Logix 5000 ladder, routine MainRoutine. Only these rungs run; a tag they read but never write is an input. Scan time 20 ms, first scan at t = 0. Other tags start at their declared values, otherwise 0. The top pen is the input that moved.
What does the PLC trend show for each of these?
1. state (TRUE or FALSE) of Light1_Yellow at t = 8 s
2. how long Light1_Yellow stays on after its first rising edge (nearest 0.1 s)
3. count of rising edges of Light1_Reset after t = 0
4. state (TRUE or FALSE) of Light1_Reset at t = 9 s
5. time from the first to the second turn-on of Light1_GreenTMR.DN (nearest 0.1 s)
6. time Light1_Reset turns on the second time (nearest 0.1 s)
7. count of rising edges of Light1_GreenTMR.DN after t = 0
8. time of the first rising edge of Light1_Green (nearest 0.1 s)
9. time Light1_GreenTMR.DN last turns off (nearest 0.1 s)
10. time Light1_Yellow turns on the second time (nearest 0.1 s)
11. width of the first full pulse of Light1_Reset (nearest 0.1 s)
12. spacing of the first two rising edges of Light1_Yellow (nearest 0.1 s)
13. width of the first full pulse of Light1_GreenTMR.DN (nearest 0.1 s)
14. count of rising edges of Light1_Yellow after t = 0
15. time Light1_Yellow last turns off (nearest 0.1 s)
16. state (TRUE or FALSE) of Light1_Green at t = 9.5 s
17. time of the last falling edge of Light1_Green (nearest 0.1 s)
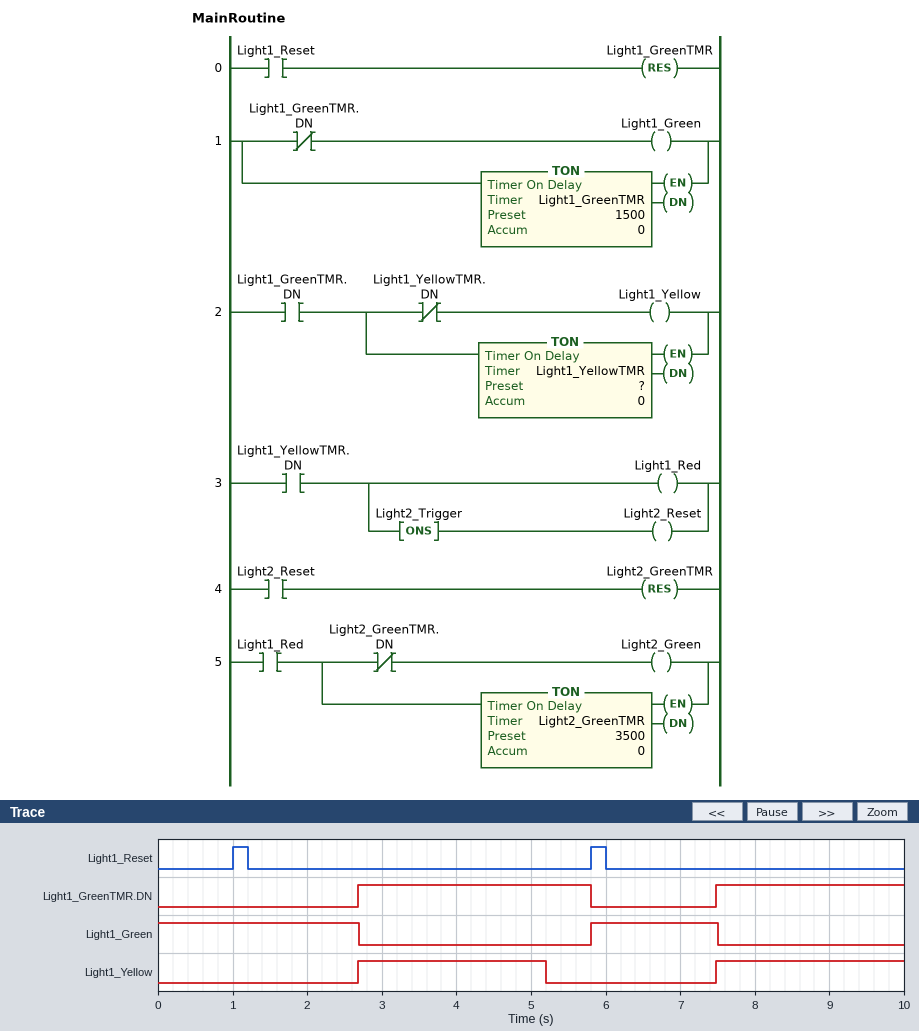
TRUE
2.5 s
2
FALSE
4.8 s
5.8 s
2
5.8 s
5.8 s
7.5 s
0.2 s
4.8 s
3.1 s
2
5.2 s
FALSE
7.5 s
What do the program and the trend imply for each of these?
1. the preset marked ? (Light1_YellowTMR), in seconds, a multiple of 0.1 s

2.5 s
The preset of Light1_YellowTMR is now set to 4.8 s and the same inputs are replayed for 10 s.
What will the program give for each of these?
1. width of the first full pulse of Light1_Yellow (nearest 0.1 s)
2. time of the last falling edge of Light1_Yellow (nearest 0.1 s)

3.1 s
5.8 s
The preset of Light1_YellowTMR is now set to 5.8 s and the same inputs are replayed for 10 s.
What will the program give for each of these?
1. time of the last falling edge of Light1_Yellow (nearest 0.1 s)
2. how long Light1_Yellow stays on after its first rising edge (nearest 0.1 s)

5.8 s
3.1 s
